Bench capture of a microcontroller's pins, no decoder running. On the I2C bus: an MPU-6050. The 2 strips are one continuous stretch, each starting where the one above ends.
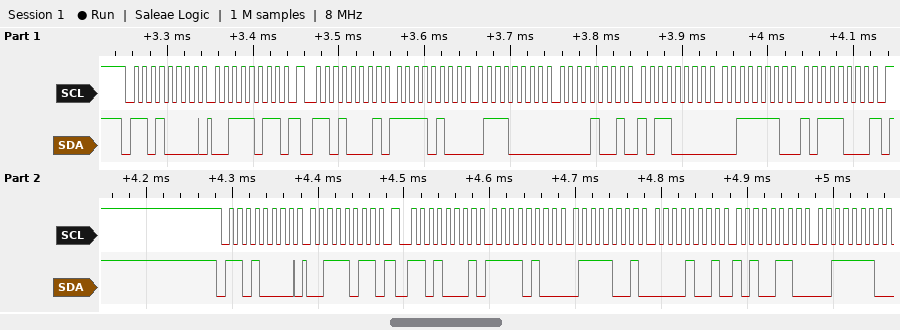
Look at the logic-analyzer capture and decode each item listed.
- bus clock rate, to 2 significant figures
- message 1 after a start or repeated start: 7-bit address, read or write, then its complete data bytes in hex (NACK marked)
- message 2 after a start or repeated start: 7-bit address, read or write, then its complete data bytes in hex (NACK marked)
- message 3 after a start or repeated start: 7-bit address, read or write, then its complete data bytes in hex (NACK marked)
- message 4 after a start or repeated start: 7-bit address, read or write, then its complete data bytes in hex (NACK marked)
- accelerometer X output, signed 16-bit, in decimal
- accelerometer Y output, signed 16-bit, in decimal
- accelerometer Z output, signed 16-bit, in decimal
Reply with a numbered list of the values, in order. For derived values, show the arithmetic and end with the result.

1. 100 kHz
2. 0x68 write: 3B
3. 0x68 read: F4 70 09 B0 3E B8 NACK
4. 0x68 write: 3B
5. 0x68 read: F4 79 09 A6 3E
6. 0xF470 = -2960
7. 0x09B0 = 2480
8. 0x3EB8 = 16056
